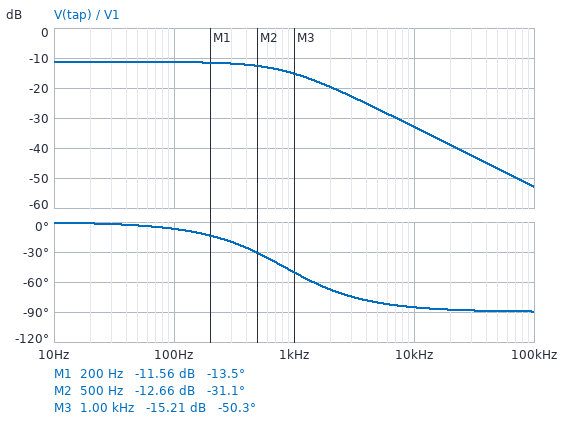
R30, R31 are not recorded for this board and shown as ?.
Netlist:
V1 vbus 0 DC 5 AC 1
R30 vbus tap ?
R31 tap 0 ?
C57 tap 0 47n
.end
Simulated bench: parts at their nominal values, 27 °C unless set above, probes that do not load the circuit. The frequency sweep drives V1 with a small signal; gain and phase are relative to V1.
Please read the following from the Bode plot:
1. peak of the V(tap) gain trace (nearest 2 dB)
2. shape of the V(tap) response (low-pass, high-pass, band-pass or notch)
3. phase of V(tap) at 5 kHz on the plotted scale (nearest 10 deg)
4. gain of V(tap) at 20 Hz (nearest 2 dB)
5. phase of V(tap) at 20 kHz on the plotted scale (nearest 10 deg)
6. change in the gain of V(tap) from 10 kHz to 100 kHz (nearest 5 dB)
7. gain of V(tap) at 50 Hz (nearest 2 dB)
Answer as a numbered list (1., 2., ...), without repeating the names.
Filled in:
1. -12 dB
2. low-pass
3. -80 deg
4. -12 dB
5. -90 deg
6. -20 dB
7. -12 dB
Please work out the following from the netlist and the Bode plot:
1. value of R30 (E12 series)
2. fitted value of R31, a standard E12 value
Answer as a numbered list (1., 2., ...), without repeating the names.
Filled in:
1. 15 kΩ
2. 5.6 kΩ
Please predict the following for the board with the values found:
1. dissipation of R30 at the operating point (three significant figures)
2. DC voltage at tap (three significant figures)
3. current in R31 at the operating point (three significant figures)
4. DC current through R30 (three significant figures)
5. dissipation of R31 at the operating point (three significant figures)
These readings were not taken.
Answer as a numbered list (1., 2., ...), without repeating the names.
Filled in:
1. 884 µW
2. 1.36 V
3. 243 µA
4. 243 µA
5. 330 µW
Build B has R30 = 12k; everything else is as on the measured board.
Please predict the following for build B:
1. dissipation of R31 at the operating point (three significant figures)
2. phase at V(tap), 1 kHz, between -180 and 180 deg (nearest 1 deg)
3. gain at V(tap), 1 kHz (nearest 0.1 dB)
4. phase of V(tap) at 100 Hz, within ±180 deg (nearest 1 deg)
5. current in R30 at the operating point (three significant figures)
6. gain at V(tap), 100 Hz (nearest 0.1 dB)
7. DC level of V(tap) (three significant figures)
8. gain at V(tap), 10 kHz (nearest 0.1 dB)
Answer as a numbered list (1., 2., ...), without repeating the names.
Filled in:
1. 452 µW
2. -48 deg
3. -13.5 dB
4. -6 deg
5. 284 µA
6. -10.0 dB
7. 1.59 V
8. -31.0 dB
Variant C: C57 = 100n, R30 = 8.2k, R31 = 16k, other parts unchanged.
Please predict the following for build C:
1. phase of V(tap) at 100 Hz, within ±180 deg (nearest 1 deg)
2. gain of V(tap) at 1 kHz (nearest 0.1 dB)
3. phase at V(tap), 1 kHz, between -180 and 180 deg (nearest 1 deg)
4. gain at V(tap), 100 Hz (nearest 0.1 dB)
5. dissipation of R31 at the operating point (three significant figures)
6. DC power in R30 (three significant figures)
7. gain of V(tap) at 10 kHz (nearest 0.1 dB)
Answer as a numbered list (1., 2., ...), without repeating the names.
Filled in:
1. -19 deg
2. -14.6 dB
3. -74 deg
4. -4.1 dB
5. 683 µW
6. 350 µW
7. -34.2 dB
